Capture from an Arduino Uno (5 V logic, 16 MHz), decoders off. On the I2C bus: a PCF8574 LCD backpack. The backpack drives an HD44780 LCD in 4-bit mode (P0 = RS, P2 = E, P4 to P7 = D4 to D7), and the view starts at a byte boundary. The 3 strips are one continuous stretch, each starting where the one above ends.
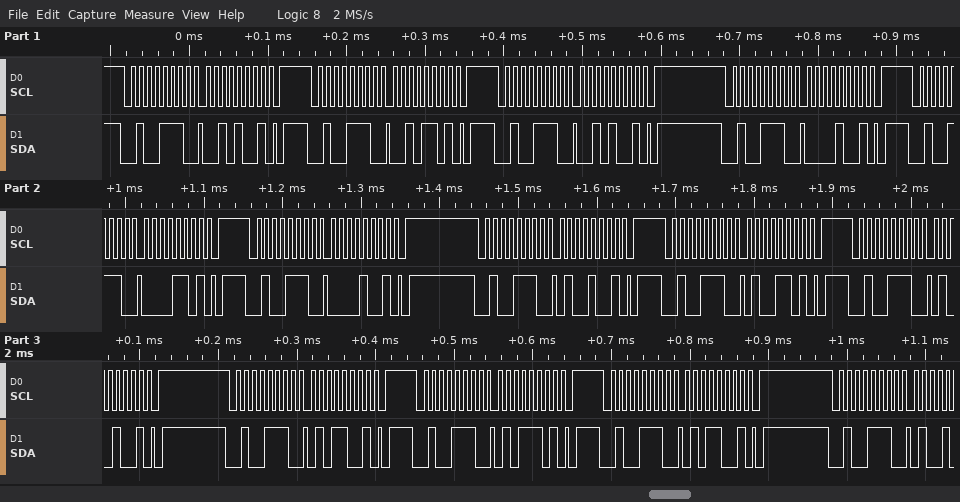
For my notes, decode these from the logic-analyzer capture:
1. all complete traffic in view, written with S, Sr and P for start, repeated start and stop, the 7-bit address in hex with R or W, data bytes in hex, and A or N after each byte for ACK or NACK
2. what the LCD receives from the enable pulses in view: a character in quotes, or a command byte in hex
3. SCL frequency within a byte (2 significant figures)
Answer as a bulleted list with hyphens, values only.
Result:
- S 27W A 29 A P S 27W A 2D A P S 27W A 29 A P S 27W A 09 A P S 27W A 0D A P S 27W A 09 A P S 27W A 49 A P S 27W A 4D A P S 27W A 49 A P S 27W A 59 A P S 27W A 5D A P S 27W A 59 A P S 27W A
- ' ' 'E'
- 100 kHz
